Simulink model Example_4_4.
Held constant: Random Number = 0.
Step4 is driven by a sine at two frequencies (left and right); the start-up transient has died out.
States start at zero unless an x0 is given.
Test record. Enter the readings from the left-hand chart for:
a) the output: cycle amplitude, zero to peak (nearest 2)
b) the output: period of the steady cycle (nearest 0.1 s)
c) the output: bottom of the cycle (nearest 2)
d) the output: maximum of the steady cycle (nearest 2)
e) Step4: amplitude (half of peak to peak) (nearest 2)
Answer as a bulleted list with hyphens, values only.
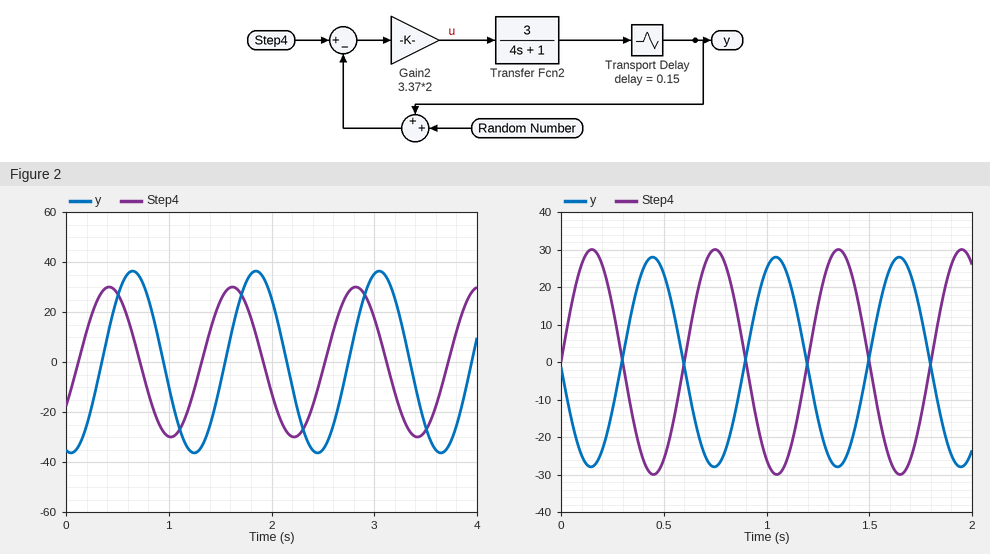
- 36
- 1.2 s
- -36
- 36
- 30
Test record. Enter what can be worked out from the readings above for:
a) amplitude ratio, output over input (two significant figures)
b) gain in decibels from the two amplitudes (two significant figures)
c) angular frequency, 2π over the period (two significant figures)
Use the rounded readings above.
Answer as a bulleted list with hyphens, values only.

- 1.2
- 1.6 dB
- 5.2 rad/s
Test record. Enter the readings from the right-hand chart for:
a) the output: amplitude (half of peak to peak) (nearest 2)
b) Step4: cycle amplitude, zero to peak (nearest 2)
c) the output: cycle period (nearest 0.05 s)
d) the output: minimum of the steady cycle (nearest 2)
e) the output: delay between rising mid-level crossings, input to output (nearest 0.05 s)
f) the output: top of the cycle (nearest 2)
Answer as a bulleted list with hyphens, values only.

- 28
- 30
- 0.60 s
- -28
- 0.30 s
- 28
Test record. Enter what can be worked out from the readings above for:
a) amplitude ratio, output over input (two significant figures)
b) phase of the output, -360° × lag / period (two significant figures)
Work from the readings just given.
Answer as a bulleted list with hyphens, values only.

- 0.93
- -180°
